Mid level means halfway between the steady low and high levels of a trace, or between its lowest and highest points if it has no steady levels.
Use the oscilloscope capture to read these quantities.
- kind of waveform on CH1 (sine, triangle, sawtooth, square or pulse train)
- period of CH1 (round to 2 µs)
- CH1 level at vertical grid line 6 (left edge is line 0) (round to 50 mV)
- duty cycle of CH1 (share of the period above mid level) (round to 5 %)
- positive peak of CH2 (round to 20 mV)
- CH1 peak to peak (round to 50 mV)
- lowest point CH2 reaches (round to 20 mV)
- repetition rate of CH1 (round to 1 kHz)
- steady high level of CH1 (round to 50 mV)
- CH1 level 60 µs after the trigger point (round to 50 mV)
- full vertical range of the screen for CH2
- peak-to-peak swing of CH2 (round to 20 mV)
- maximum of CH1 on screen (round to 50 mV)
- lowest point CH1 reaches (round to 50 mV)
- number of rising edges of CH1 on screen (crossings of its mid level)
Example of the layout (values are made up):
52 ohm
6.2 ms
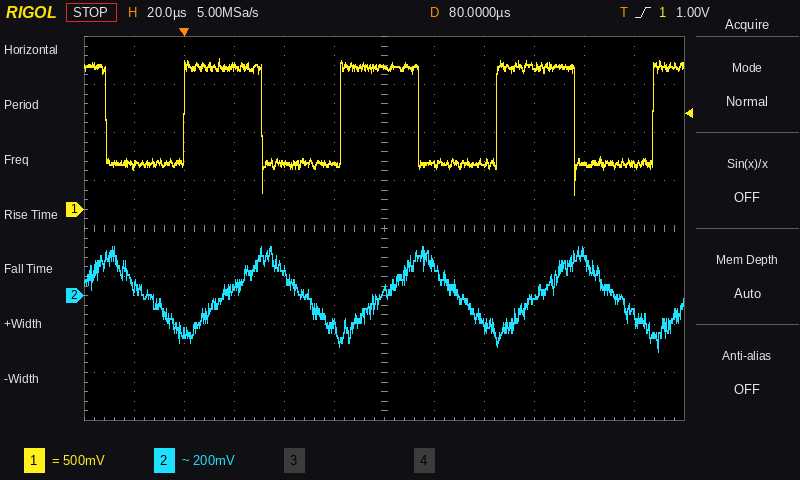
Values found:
square
62 µs
1.50 V
50 %
200 mV
1.40 V
-240 mV
16 kHz
1.50 V
450 mV
1.6 V
440 mV
1.55 V
150 mV
4
